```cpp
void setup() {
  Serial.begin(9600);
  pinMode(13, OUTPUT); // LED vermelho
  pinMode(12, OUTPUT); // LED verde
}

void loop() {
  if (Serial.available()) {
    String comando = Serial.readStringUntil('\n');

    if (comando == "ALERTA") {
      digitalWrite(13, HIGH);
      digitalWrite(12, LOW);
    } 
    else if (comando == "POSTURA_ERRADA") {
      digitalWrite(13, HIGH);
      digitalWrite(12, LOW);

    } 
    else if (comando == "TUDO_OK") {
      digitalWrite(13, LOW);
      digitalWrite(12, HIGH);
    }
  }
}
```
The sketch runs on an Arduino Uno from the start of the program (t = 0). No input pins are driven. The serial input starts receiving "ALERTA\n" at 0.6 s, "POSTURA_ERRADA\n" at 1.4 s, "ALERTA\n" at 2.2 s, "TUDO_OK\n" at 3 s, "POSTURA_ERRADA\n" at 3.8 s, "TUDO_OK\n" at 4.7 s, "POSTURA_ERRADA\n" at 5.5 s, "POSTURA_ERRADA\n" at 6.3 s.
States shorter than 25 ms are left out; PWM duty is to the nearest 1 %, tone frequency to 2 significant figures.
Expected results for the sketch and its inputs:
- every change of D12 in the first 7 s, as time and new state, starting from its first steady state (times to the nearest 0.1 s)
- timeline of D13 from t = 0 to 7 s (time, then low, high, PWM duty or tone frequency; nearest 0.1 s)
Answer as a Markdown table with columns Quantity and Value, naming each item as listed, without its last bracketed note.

| Quantity | Value |
|---|---|
| every change of D12 in the first 7 s, as time and new state, starting from its first steady state | 0 s low; 3 s high; 3.8 s low; 4.7 s high; 5.5 s low |
| timeline of D13 from t = 0 to 7 s | 0 s low; 0.6 s high; 3 s low; 3.8 s high; 4.7 s low; 5.5 s high |
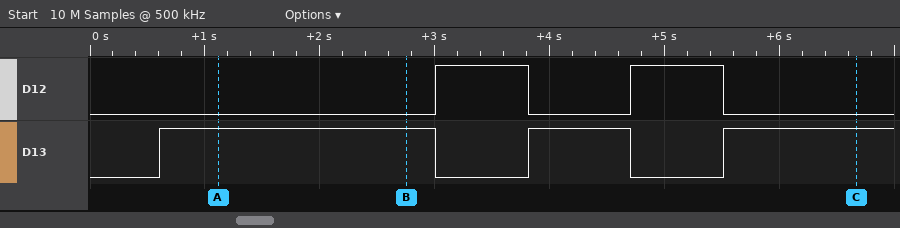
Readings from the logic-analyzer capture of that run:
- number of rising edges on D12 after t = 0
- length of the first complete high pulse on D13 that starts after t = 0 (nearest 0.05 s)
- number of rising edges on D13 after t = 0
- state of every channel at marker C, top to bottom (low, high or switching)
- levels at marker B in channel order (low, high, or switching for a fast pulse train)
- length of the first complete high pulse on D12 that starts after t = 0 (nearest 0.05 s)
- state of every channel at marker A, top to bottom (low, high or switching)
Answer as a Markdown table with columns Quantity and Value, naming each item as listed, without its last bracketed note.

| Quantity | Value |
|---|---|
| number of rising edges on D12 after t = 0 | 2 |
| length of the first complete high pulse on D13 that starts after t = 0 | 2.40 s |
| number of rising edges on D13 after t = 0 | 3 |
| state of every channel at marker C, top to bottom | D12 low, D13 high |
| levels at marker B in channel order | D12 low, D13 high |
| length of the first complete high pulse on D12 that starts after t = 0 | 0.80 s |
| state of every channel at marker A, top to bottom | D12 low, D13 high |
